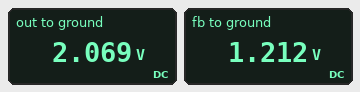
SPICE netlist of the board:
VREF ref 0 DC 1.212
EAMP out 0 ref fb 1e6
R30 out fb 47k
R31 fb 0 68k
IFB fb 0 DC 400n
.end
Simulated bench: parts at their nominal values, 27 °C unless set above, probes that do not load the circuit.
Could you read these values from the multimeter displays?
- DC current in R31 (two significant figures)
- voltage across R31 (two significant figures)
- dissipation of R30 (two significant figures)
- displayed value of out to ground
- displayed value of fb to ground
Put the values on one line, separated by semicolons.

18 µA; 1.2 V; 16 µW; 2.069 V; 1.212 V
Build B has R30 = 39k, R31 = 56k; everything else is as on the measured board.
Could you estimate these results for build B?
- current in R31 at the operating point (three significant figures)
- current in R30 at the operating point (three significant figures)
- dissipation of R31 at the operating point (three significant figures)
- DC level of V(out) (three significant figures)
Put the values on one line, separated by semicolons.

21.6 µA; 22.0 µA; 26.2 µW; 2.07 V
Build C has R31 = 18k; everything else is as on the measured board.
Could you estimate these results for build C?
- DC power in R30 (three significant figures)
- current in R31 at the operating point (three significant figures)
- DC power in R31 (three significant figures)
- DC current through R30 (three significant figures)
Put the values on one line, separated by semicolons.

216 µW; 67.3 µA; 81.6 µW; 67.7 µA
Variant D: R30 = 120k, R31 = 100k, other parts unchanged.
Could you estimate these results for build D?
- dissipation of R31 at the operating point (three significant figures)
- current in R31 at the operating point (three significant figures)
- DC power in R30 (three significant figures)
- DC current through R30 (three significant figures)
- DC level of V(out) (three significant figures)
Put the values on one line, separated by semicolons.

14.7 µW; 12.1 µA; 18.8 µW; 12.5 µA; 2.71 V
